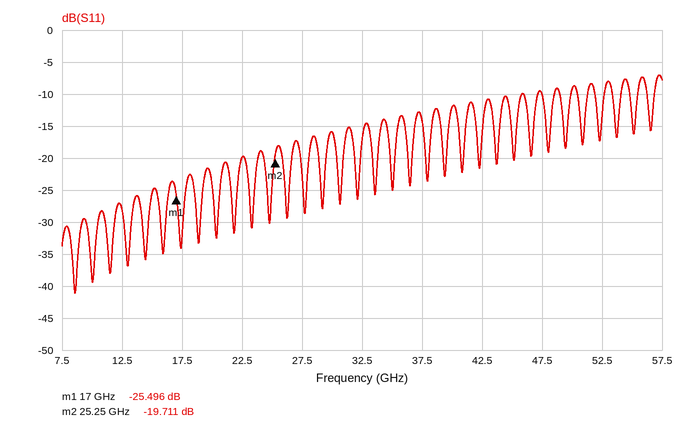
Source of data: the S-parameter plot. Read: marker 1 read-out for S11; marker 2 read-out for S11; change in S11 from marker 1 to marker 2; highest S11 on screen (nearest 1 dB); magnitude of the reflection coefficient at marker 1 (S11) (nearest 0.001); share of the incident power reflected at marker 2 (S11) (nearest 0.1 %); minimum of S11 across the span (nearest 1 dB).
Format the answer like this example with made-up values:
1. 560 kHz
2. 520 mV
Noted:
1. -25.496 dB
2. -19.711 dB
3. 5.785 dB
4. -7 dB
5. 0.053
6. 1.1 %
7. -41 dB
